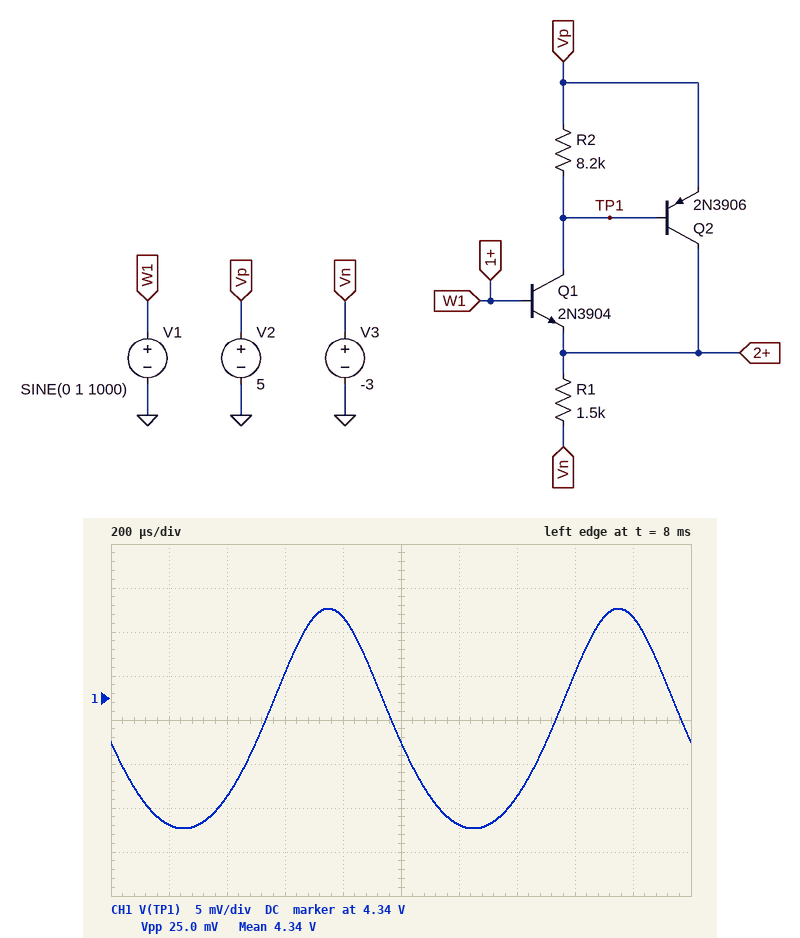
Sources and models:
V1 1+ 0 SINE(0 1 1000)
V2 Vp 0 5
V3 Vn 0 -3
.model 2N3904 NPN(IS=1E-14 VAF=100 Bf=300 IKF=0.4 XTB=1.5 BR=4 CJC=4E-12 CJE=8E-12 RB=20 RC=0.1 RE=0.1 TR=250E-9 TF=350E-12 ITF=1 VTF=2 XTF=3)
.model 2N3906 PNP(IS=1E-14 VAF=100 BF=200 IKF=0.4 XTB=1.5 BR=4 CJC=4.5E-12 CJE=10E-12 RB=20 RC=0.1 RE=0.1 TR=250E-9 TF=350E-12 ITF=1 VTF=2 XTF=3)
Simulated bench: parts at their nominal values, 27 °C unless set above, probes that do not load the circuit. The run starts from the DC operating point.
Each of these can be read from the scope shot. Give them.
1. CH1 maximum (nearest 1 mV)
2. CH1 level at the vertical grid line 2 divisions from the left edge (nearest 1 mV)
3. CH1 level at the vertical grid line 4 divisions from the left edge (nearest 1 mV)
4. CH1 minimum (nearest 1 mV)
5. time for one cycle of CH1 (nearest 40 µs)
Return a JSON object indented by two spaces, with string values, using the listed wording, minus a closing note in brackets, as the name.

{
  "CH1 maximum": "4.350 V",
  "CH1 level at the vertical grid line 2 divisions from the left edge": "4.329 V",
  "CH1 level at the vertical grid line 4 divisions from the left edge": "4.349 V",
  "CH1 minimum": "4.325 V",
  "time for one cycle of CH1": "1.00 ms"
}
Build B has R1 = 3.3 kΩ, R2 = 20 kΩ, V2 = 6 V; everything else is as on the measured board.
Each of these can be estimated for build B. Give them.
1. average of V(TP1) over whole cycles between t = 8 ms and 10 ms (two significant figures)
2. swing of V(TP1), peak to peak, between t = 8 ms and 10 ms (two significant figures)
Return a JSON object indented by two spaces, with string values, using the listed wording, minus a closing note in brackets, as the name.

{
  "average of V(TP1) over whole cycles between t = 8 ms and 10 ms": "5.4 V",
  "swing of V(TP1), peak to peak, between t = 8 ms and 10 ms": "24 mV"
}
